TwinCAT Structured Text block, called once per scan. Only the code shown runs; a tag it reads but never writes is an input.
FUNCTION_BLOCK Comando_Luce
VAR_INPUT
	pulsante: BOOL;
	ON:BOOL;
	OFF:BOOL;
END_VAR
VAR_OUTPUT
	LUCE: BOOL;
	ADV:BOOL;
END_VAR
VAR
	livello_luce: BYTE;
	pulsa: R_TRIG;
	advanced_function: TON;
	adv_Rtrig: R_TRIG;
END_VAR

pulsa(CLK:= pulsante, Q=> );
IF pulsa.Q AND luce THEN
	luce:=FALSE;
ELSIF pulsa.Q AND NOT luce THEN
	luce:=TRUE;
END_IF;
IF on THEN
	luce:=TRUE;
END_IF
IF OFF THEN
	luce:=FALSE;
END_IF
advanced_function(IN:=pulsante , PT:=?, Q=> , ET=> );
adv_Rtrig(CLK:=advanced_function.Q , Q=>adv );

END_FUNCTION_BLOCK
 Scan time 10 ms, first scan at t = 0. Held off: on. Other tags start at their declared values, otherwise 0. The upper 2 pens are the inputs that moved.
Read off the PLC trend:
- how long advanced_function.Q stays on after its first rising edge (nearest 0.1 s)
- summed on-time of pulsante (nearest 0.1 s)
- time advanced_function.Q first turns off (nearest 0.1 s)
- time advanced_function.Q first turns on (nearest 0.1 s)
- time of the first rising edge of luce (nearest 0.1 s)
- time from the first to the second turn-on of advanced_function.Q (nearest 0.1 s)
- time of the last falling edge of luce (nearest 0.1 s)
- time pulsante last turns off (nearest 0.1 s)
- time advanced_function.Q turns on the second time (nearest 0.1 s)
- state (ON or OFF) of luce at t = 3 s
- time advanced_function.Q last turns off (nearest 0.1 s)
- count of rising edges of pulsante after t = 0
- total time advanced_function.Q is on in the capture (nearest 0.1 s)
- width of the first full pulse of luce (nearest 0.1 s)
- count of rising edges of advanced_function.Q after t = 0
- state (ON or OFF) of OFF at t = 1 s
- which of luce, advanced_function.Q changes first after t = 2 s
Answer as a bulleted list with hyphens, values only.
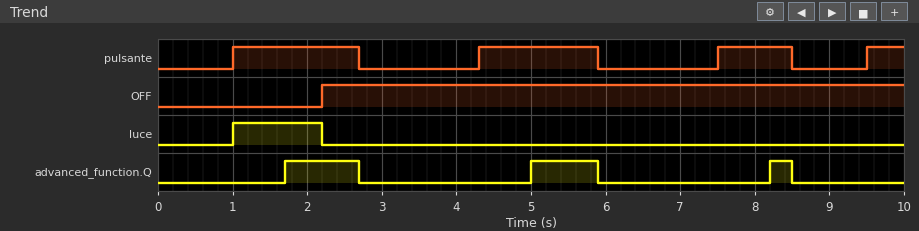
- 1.0 s
- 4.8 s
- 2.7 s
- 1.7 s
- 1.0 s
- 3.3 s
- 2.2 s
- 8.5 s
- 5.0 s
- OFF
- 8.5 s
- 4
- 2.2 s
- 1.2 s
- 3
- OFF
- luce
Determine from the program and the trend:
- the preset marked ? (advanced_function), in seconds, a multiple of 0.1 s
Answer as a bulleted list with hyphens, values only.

- 0.7 s
